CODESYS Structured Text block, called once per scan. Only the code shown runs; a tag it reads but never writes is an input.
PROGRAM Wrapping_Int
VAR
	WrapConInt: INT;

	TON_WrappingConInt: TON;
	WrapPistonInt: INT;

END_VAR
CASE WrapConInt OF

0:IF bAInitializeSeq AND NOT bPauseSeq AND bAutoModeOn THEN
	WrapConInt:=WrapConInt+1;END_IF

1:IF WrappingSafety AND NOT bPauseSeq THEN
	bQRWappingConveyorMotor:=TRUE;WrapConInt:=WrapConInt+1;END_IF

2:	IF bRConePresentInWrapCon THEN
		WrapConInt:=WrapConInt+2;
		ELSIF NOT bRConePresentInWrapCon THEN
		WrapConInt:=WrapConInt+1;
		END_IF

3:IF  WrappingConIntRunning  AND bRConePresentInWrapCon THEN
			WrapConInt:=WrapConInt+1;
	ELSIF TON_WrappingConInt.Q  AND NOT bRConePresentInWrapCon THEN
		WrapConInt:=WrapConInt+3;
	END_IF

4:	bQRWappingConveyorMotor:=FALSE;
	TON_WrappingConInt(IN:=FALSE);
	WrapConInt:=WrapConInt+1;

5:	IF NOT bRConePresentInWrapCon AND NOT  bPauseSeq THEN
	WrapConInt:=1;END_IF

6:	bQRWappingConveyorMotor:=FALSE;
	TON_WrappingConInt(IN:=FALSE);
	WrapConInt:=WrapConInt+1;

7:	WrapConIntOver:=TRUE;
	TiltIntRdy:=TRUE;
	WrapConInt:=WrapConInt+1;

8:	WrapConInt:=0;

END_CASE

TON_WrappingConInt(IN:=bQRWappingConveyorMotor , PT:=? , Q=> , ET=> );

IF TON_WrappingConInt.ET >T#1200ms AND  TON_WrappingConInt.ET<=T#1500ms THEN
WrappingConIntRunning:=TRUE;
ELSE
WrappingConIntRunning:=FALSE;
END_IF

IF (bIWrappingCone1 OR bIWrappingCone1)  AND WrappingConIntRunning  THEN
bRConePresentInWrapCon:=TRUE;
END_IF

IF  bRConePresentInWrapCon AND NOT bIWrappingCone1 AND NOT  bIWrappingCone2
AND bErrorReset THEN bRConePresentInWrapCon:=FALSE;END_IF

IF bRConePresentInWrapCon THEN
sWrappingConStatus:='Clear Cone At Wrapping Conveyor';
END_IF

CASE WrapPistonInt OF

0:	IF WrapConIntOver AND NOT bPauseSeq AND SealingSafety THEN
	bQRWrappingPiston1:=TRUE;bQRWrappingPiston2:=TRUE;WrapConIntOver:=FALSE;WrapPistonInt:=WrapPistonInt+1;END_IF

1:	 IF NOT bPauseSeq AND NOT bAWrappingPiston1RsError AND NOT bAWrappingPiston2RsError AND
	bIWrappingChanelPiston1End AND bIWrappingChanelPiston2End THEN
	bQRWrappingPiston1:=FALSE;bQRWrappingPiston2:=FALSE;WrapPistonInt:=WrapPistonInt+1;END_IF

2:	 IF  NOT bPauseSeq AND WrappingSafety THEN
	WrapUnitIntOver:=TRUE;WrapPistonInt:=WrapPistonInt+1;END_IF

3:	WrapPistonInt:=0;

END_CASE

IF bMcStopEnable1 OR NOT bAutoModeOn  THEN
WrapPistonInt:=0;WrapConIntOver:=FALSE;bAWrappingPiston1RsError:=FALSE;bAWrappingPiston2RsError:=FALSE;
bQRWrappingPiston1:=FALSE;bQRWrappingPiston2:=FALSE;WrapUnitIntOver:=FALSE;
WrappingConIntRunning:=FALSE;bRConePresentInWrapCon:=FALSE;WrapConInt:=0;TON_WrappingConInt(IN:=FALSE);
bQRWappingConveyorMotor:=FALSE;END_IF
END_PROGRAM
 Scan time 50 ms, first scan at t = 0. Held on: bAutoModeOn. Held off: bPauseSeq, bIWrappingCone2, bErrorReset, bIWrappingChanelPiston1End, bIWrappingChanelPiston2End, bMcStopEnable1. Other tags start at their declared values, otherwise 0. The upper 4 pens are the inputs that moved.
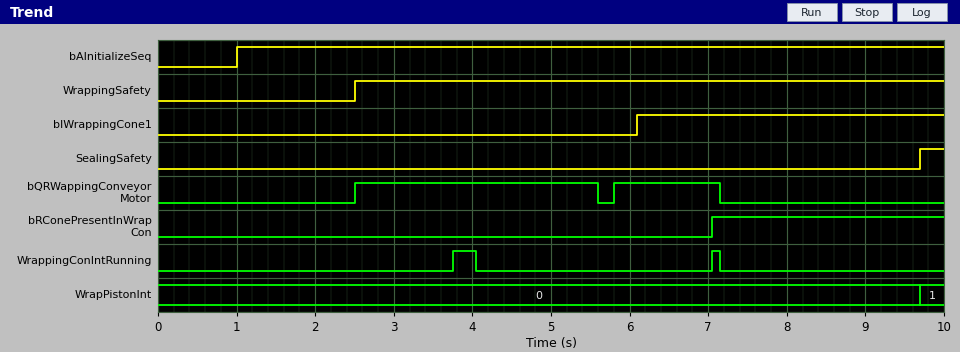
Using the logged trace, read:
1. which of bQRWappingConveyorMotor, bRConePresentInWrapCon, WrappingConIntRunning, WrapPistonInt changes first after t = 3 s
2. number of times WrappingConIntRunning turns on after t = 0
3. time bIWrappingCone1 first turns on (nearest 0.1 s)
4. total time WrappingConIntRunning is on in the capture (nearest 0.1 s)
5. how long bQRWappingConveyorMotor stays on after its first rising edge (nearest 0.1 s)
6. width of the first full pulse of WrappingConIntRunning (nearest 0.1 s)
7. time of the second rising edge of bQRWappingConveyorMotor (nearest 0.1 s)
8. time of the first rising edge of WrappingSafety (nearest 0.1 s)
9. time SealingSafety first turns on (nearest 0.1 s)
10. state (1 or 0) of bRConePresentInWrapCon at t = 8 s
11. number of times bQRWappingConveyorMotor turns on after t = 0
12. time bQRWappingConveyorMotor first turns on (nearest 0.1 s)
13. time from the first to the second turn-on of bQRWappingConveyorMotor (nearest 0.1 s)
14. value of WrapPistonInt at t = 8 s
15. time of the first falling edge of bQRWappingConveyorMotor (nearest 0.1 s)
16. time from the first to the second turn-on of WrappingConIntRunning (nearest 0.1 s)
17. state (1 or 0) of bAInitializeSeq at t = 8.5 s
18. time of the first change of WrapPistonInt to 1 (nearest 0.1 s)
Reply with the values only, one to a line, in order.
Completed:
WrappingConIntRunning
2
6.1 s
0.4 s
3.1 s
0.3 s
5.8 s
2.5 s
9.7 s
1
2
2.5 s
3.3 s
0
5.6 s
3.3 s
1
9.7 s
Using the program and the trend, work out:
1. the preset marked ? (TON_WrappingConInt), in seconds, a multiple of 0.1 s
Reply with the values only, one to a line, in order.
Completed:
3.0 s
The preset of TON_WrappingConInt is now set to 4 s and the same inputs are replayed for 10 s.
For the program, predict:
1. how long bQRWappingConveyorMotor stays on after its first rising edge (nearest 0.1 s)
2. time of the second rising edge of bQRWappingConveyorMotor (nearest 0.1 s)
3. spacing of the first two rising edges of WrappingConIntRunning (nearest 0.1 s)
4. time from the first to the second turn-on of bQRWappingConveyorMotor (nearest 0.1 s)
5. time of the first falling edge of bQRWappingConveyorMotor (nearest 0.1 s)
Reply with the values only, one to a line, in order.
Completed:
4.1 s
6.8 s
4.3 s
4.3 s
6.6 s
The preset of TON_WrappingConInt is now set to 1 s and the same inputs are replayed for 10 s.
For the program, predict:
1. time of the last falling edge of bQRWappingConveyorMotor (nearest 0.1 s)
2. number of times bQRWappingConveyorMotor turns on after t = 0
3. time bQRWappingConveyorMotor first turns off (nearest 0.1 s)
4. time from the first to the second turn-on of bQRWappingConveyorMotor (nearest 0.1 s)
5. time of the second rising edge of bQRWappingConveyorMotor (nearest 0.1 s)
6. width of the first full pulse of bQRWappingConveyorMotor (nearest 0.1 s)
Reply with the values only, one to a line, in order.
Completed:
8.8 s
6
3.6 s
1.3 s
3.8 s
1.1 s
